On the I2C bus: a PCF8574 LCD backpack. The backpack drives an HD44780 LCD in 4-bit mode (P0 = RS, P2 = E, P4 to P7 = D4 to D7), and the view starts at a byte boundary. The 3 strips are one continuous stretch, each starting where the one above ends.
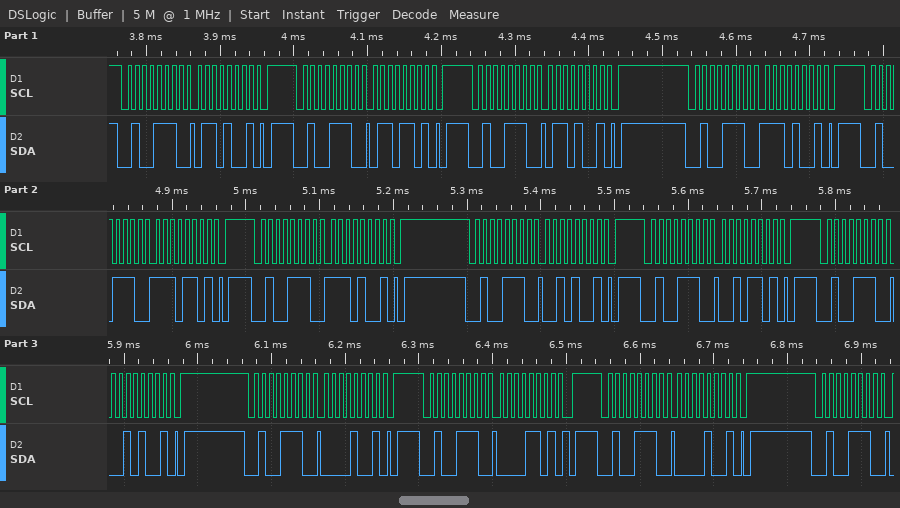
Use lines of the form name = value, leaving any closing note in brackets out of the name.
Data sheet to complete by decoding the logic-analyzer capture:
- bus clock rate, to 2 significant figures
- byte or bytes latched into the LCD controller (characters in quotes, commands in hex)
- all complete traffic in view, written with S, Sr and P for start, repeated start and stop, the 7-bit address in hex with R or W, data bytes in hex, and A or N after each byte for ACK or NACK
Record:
bus clock rate, to 2 significant figures = 100 kHz
byte or bytes latched into the LCD controller = 'n' ' '
all complete traffic in view, written with S, Sr and P for start, repeated start and stop, the 7-bit address in hex with R or W, data bytes in hex, and A or N after each byte for ACK or NACK = S 27W A 69 A P S 27W A 6D A P S 27W A 69 A P S 27W A E9 A P S 27W A ED A P S 27W A E9 A P S 27W A 29 A P S 27W A 2D A P S 27W A 29 A P S 27W A 09 A P S 27W A 0D A P S 27W A 09 A P S 27W A
